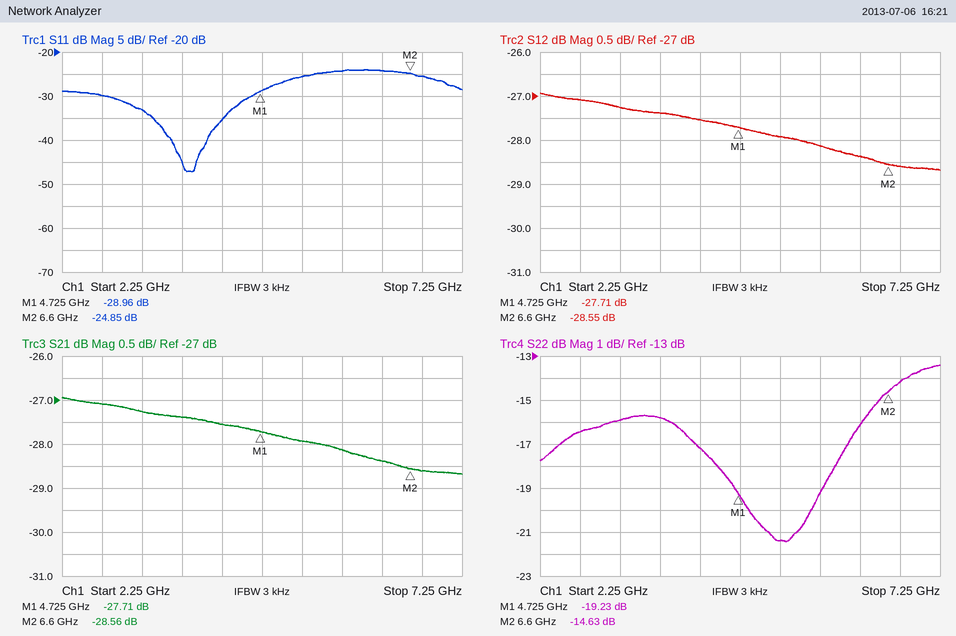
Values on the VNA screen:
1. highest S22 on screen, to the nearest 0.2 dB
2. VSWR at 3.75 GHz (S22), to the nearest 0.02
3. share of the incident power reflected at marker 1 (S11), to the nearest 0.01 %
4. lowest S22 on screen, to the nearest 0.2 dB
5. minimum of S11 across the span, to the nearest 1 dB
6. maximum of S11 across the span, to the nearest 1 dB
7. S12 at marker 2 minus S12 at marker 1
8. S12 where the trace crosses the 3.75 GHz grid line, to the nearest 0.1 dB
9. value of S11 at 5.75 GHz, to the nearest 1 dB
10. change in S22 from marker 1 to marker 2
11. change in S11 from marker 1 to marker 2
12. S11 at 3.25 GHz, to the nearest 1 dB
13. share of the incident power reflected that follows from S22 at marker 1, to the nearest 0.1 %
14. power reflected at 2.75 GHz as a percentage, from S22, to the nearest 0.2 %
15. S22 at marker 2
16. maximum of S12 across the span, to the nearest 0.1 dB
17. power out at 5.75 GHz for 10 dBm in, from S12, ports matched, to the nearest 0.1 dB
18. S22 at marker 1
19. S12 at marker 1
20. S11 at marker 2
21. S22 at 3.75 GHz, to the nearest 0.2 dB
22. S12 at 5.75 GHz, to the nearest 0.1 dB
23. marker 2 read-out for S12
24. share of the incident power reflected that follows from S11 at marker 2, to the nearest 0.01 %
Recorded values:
-13.4 dB
1.38
0.13 %
-21.4 dB
-47 dB
-24 dB
-0.84 dB
-27.4 dB
-24 dB
4.60 dB
4.11 dB
-33 dB
1.2 %
2.2 %
-14.63 dB
-26.9 dB
-18.1 dBm
-19.23 dB
-27.71 dB
-24.85 dB
-15.8 dB
-28.1 dB
-28.55 dB
0.33 %
